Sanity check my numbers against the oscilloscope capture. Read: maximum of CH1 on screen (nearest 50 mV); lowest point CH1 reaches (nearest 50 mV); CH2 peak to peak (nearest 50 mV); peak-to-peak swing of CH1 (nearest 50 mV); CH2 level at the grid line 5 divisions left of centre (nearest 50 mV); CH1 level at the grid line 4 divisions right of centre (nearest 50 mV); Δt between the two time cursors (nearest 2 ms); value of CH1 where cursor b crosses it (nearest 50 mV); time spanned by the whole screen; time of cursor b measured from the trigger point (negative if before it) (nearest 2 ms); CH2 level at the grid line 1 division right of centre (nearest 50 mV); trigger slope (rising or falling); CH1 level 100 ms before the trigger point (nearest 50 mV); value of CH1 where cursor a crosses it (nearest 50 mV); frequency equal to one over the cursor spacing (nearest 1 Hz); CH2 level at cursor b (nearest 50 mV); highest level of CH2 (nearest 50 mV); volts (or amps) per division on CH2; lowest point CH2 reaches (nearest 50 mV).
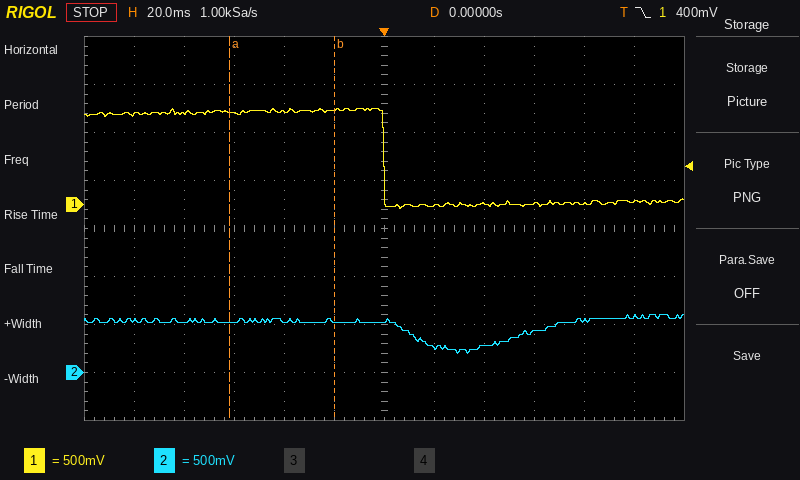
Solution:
1.00 V
-50 mV
400 mV
1.05 V
550 mV
0 mV
42 ms
1.00 V
240 ms
-20 ms
250 mV
falling
950 mV
950 mV
24 Hz
550 mV
600 mV
500 mV
200 mV
